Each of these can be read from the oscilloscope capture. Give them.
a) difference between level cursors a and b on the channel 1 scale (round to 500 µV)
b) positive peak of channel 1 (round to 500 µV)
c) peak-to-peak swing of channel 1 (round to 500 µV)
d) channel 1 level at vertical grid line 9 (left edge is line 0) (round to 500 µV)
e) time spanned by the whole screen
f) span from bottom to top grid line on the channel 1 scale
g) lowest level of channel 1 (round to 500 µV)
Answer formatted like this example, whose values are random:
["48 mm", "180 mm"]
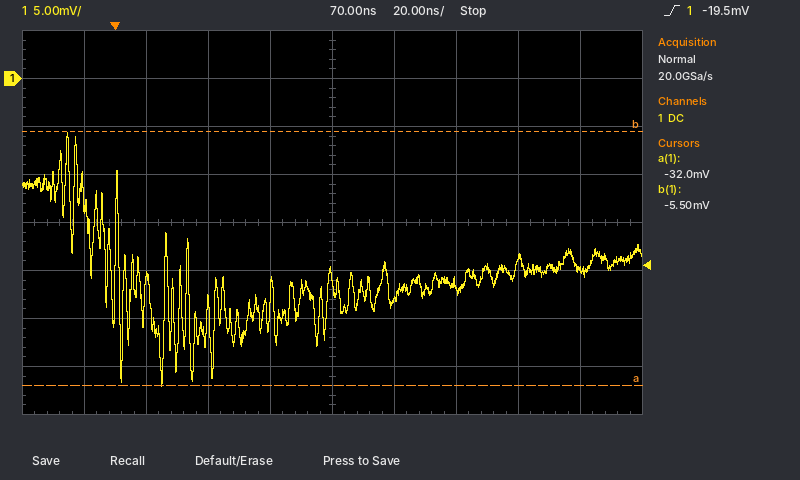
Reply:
["26.5 mV", "-5.5 mV", "26.5 mV", "-20.0 mV", "200 ns", "40 mV", "-32.0 mV"]
